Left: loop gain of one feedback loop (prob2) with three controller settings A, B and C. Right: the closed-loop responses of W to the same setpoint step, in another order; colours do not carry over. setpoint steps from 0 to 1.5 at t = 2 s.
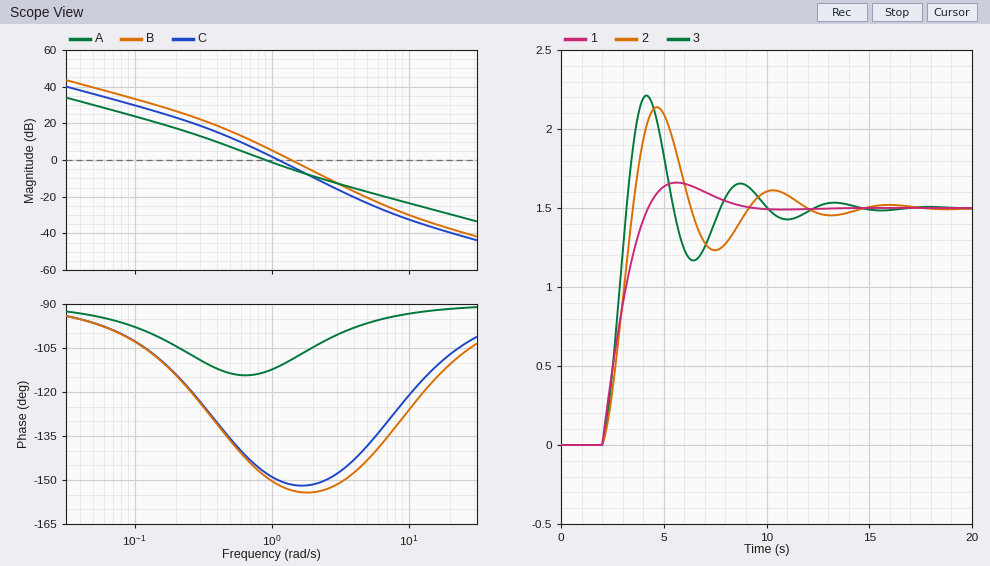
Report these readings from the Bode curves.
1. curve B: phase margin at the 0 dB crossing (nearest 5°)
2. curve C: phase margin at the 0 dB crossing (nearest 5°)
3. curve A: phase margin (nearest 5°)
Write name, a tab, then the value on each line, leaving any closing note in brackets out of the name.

curve B: phase margin at the 0 dB crossing	25°
curve C: phase margin at the 0 dB crossing	30°
curve A: phase margin	65°
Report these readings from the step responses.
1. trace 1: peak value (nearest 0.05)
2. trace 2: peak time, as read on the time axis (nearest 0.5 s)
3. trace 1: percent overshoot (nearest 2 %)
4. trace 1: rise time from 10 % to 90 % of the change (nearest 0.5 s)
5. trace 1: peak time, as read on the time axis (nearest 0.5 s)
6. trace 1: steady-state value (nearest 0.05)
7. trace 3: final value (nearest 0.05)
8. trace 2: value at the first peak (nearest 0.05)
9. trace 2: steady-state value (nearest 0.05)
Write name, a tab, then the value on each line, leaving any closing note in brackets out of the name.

trace 1: peak value	1.65
trace 2: peak time, as read on the time axis	4.5 s
trace 1: percent overshoot	10 %
trace 1: rise time from 10 % to 90 % of the change	1.5 s
trace 1: peak time, as read on the time axis	5.5 s
trace 1: steady-state value	1.50
trace 3: final value	1.50
trace 2: value at the first peak	2.15
trace 2: steady-state value	1.50
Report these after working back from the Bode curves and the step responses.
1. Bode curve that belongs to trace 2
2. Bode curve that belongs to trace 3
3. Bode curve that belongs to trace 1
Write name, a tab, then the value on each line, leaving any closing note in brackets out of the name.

Bode curve that belongs to trace 2	C
Bode curve that belongs to trace 3	B
Bode curve that belongs to trace 1	A
